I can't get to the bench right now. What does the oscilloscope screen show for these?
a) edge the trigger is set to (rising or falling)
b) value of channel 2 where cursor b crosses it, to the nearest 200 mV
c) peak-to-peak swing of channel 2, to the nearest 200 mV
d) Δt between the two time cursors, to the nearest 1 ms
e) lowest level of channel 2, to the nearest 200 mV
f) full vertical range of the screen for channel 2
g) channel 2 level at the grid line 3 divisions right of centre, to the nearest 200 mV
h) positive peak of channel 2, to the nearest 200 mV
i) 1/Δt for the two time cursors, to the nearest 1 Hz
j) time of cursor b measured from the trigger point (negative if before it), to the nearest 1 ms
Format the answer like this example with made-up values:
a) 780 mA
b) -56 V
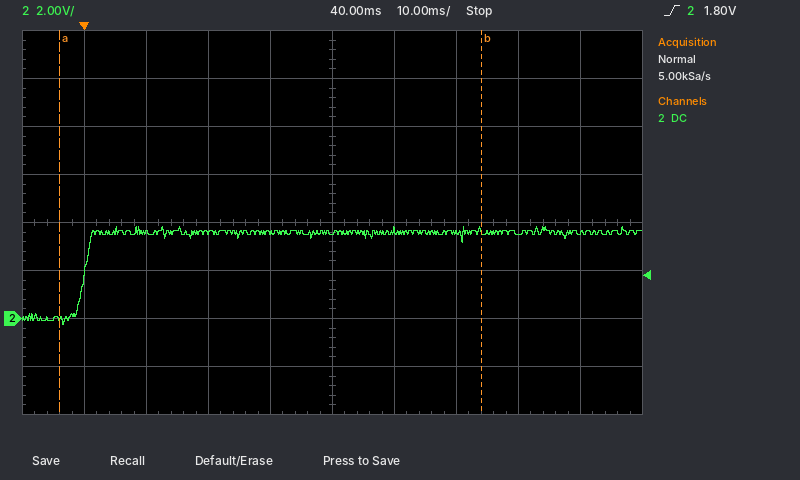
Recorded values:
a) rising
b) 3.6 V
c) 4.0 V
d) 68 ms
e) -200 mV
f) 16 V
g) 3.6 V
h) 3.8 V
i) 15 Hz
j) +64 ms
